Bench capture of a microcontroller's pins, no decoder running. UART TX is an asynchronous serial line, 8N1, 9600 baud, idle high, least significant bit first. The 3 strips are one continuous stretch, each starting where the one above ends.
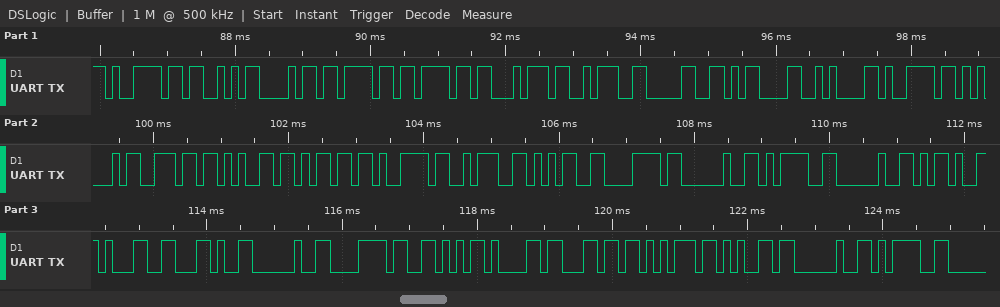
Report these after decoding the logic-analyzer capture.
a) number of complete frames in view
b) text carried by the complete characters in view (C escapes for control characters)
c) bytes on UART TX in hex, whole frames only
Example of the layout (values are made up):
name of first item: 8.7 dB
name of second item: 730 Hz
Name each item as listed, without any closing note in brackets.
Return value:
number of complete frames in view: 34
text carried by the complete characters in view: "yShoot:0\r\nyEnemy:5x = -1, xValue ="
bytes on UART TX in hex, whole frames only: 79 53 68 6F 6F 74 3A 30 0D 0A 79 45 6E 65 6D 79 3A 35 78 20 3D 20 2D 31 2C 20 78 56 61 6C 75 65 20 3D
